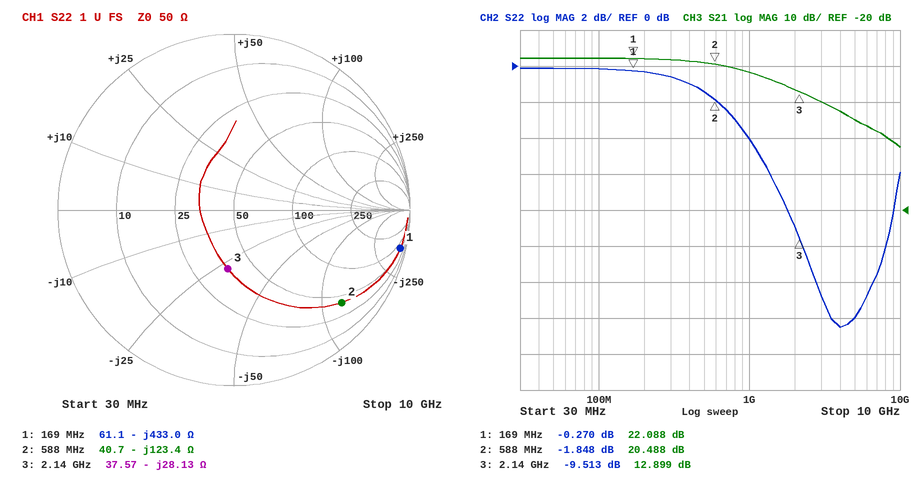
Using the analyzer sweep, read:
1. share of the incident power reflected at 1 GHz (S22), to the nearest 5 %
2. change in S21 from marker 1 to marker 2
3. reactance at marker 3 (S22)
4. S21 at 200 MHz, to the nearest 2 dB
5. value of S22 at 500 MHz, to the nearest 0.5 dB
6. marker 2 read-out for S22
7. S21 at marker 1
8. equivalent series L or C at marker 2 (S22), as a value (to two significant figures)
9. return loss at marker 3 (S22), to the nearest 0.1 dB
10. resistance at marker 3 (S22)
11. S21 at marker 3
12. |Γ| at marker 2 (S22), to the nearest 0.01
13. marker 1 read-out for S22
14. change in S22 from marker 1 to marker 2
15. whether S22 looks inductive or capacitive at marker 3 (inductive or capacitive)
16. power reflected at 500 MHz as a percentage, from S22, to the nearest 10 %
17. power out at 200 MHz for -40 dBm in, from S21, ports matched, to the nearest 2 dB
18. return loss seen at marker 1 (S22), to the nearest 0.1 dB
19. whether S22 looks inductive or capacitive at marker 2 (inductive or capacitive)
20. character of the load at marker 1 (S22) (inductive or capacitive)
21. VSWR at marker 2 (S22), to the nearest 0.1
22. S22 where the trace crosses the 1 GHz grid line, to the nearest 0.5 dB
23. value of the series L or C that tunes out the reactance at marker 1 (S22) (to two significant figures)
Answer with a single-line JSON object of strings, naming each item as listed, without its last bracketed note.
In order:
{"share of the incident power reflected at 1 GHz (S22), to the nearest 5 %": "40 %", "change in S21 from marker 1 to marker 2": "-1.600 dB", "reactance at marker 3": "-28.13 Ω", "S21 at 200 MHz, to the nearest 2 dB": "22 dB", "value of S22 at 500 MHz, to the nearest 0.5 dB": "-1.5 dB", "marker 2 read-out for S22": "-1.848 dB", "S21 at marker 1": "22.088 dB", "equivalent series L or C at marker 2 (S22), as a value": "2.2 pF", "return loss at marker 3 (S22), to the nearest 0.1 dB": "9.5 dB", "resistance at marker 3": "37.57 Ω", "S21 at marker 3": "12.899 dB", "|Γ| at marker 2 (S22), to the nearest 0.01": "0.81", "marker 1 read-out for S22": "-0.270 dB", "change in S22 from marker 1 to marker 2": "-1.578 dB", "whether S22 looks inductive or capacitive at marker 3": "capacitive", "power reflected at 500 MHz as a percentage, from S22, to the nearest 10 %": "70 %", "power out at 200 MHz for -40 dBm in, from S21, ports matched, to the nearest 2 dB": "-18 dBm", "return loss seen at marker 1 (S22), to the nearest 0.1 dB": "0.3 dB", "whether S22 looks inductive or capacitive at marker 2": "capacitive", "character of the load at marker 1 (S22)": "capacitive", "VSWR at marker 2 (S22), to the nearest 0.1": "9.4", "S22 where the trace crosses the 1 GHz grid line, to the nearest 0.5 dB": "-4.0 dB", "value of the series L or C that tunes out the reactance at marker 1 (S22)": "410 nH"}
